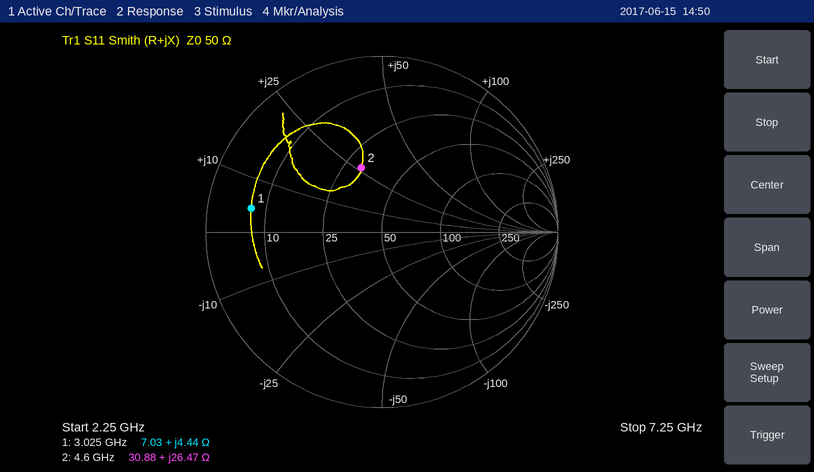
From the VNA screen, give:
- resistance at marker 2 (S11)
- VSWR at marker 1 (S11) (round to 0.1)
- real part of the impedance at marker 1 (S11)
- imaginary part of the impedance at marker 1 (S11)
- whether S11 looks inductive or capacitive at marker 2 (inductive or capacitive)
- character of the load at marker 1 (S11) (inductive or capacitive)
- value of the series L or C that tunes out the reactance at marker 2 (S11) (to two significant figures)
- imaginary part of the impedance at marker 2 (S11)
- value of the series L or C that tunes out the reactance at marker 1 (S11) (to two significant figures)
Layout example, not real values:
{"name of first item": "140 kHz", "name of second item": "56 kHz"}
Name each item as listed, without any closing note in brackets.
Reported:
{"resistance at marker 2": "30.88 Ω", "VSWR at marker 1 (S11)": "7.2", "real part of the impedance at marker 1": "7.03 Ω", "imaginary part of the impedance at marker 1": "+4.44 Ω", "whether S11 looks inductive or capacitive at marker 2": "inductive", "character of the load at marker 1 (S11)": "inductive", "value of the series L or C that tunes out the reactance at marker 2 (S11)": "1.3 pF", "imaginary part of the impedance at marker 2": "+26.47 Ω", "value of the series L or C that tunes out the reactance at marker 1 (S11)": "12 pF"}
